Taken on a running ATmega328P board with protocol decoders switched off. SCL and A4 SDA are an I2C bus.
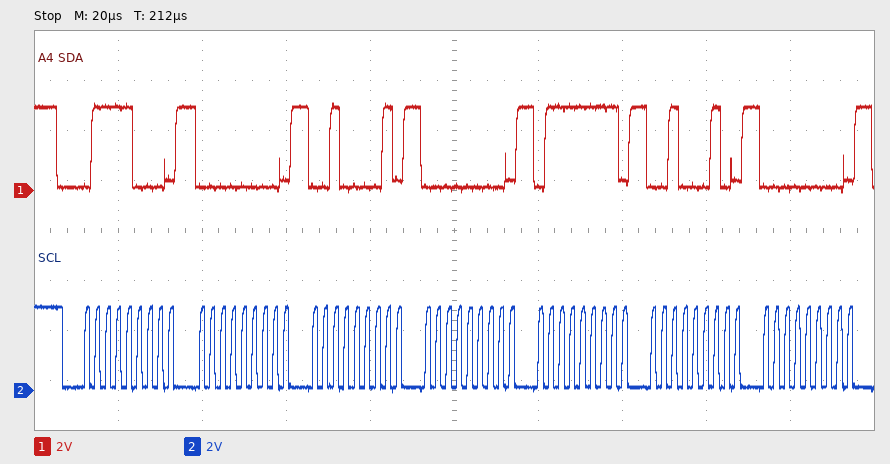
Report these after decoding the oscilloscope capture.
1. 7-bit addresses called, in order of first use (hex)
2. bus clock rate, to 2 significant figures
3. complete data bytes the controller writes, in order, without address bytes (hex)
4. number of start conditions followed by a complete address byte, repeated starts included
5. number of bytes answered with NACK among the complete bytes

0x3C
400 kHz
00 21 00 7F 22 00
1
0
